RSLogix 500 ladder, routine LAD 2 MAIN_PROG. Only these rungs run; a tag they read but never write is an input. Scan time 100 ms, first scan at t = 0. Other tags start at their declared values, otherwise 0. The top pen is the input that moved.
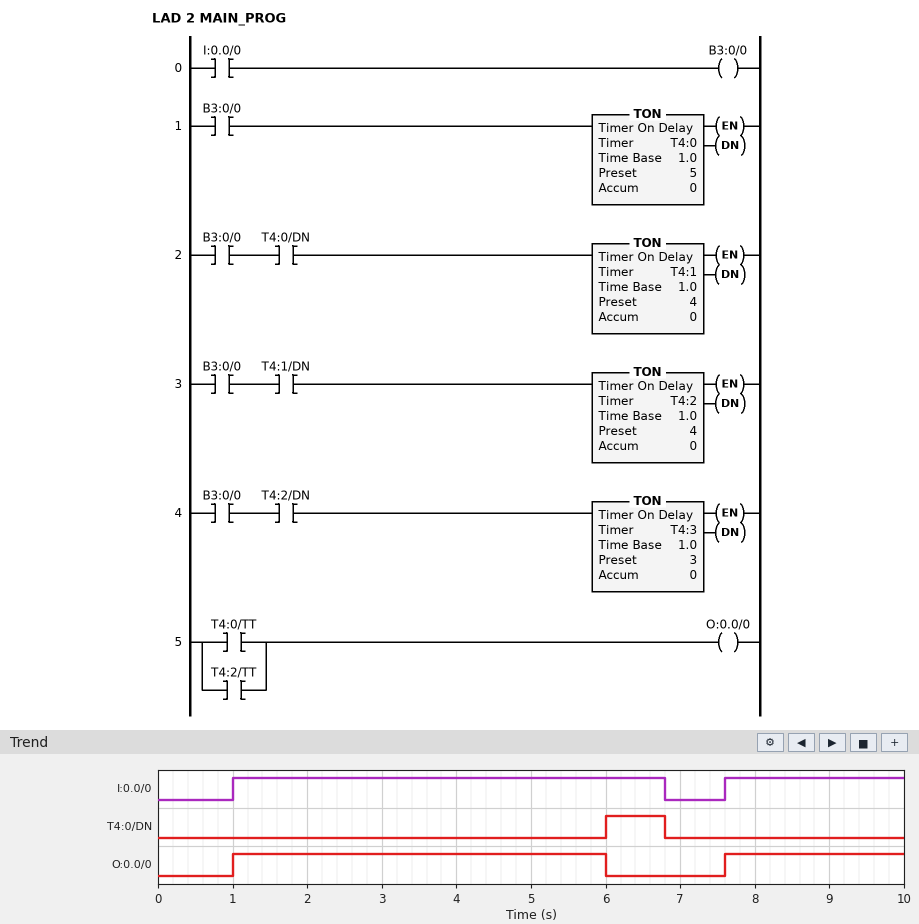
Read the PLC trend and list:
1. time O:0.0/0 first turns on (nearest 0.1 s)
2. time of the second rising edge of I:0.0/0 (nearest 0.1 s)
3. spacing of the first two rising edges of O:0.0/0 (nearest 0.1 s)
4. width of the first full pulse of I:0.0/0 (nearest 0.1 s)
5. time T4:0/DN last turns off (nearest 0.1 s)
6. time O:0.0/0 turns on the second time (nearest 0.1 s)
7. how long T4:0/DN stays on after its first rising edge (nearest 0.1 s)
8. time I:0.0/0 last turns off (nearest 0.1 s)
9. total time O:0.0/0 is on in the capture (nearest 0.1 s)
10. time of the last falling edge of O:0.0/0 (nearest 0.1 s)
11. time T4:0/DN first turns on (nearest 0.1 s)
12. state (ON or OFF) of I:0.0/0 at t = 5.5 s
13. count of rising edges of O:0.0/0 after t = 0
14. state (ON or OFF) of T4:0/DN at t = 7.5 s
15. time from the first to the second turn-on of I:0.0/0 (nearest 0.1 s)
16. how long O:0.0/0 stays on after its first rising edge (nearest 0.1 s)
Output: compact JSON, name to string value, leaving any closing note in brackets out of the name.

{"time O:0.0/0 first turns on": "1.0 s", "time of the second rising edge of I:0.0/0": "7.6 s", "spacing of the first two rising edges of O:0.0/0": "6.6 s", "width of the first full pulse of I:0.0/0": "5.8 s", "time T4:0/DN last turns off": "6.8 s", "time O:0.0/0 turns on the second time": "7.6 s", "how long T4:0/DN stays on after its first rising edge": "0.8 s", "time I:0.0/0 last turns off": "6.8 s", "total time O:0.0/0 is on in the capture": "7.4 s", "time of the last falling edge of O:0.0/0": "6.0 s", "time T4:0/DN first turns on": "6.0 s", "state (ON or OFF) of I:0.0/0 at t = 5.5 s": "ON", "count of rising edges of O:0.0/0 after t = 0": "2", "state (ON or OFF) of T4:0/DN at t = 7.5 s": "OFF", "time from the first to the second turn-on of I:0.0/0": "6.6 s", "how long O:0.0/0 stays on after its first rising edge": "5.0 s"}
